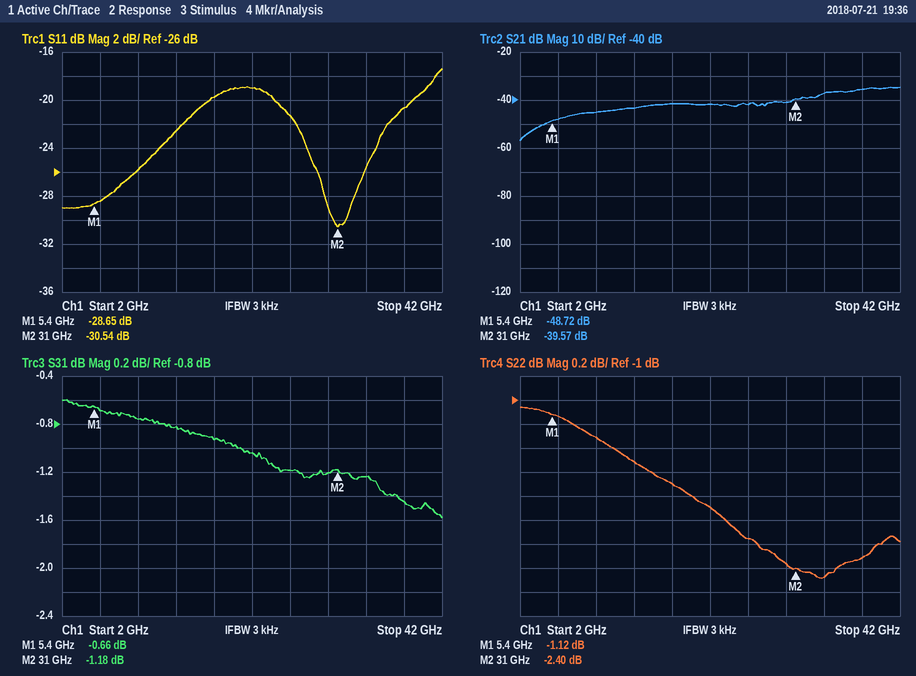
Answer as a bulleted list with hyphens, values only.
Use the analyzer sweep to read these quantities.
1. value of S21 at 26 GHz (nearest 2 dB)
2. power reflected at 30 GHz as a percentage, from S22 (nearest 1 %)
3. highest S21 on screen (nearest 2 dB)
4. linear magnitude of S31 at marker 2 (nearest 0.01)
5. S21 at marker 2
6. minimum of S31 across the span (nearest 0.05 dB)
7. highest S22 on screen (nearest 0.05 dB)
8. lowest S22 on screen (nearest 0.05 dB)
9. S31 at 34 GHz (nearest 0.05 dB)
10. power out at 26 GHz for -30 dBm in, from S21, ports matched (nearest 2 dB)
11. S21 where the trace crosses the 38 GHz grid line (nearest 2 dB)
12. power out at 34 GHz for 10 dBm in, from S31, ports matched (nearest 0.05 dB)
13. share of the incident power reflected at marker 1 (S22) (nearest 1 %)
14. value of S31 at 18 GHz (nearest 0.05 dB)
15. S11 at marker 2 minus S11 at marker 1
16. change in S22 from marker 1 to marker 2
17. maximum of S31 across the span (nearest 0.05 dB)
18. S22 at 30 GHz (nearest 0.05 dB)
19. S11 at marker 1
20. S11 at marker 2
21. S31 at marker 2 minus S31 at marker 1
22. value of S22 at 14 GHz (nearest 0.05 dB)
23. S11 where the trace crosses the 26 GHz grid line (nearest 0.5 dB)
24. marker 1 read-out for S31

- -42 dB
- 58 %
- -34 dB
- 0.87
- -39.57 dB
- -1.60 dB
- -1.05 dB
- -2.50 dB
- -1.25 dB
- -72 dBm
- -36 dB
- 8.75 dBm
- 77 %
- -0.95 dB
- -1.89 dB
- -1.28 dB
- -0.60 dB
- -2.35 dB
- -28.65 dB
- -30.54 dB
- -0.52 dB
- -1.50 dB
- -21.5 dB
- -0.66 dB
